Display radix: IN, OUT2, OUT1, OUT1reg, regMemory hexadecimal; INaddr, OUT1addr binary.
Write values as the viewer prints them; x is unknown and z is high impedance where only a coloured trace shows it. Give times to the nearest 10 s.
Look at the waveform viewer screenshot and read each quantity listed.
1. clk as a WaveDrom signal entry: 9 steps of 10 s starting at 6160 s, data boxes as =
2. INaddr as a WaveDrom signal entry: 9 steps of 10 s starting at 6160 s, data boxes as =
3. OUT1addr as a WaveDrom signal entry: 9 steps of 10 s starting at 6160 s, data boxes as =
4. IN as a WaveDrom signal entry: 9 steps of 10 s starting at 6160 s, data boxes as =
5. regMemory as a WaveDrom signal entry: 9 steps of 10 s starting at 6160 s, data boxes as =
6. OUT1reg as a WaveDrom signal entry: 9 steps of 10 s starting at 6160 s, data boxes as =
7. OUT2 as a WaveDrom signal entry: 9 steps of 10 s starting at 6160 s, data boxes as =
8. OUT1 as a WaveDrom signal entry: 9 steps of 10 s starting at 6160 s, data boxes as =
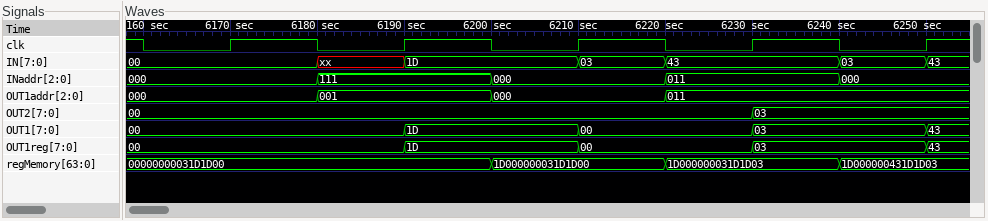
{name: 'clk', wave: '010101010'}
{name: 'INaddr', wave: '=.=.=.=.=', data: '000 111 000 011 000'}
{name: 'OUT1addr', wave: '=.=.=.=..', data: '000 001 000 011'}
{name: 'IN', wave: '=.x=.==.=', data: '00 1D 03 43 03'}
{name: 'regMemory', wave: '=...=.=.=', data: '00000000031D1D00 1D000000031D1D00 1D000000031D1D03 1D000000431D1D03'}
{name: 'OUT1reg', wave: '=..=.=.=.', data: '00 1D 00 03'}
{name: 'OUT2', wave: '=......=.', data: '00 03'}
{name: 'OUT1', wave: '=..=.=.=.', data: '00 1D 00 03'}
